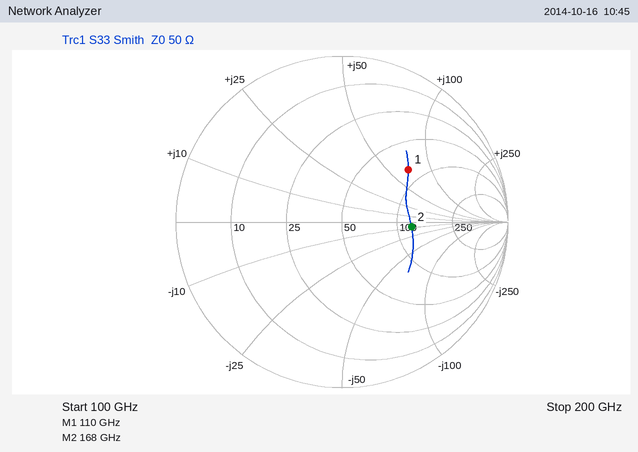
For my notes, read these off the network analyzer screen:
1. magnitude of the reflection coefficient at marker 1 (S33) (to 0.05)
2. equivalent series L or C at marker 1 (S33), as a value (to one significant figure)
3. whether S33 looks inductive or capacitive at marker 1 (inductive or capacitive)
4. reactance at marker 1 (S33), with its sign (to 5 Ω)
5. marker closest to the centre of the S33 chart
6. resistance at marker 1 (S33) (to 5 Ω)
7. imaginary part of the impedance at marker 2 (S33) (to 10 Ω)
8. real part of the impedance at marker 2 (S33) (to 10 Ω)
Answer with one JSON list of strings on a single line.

["0.50", "100 pH", "inductive", "+70 Ω", "marker 2", "80 Ω", "-10 Ω", "120 Ω"]
